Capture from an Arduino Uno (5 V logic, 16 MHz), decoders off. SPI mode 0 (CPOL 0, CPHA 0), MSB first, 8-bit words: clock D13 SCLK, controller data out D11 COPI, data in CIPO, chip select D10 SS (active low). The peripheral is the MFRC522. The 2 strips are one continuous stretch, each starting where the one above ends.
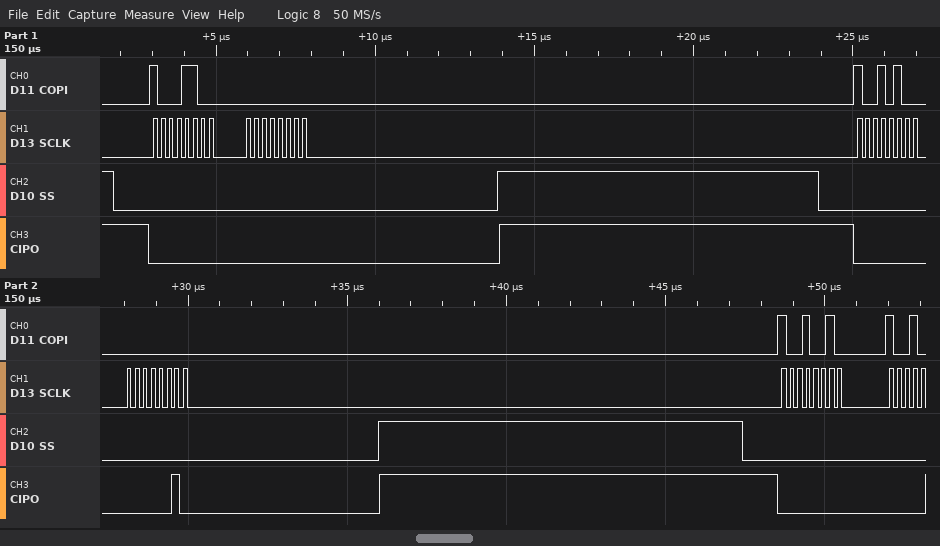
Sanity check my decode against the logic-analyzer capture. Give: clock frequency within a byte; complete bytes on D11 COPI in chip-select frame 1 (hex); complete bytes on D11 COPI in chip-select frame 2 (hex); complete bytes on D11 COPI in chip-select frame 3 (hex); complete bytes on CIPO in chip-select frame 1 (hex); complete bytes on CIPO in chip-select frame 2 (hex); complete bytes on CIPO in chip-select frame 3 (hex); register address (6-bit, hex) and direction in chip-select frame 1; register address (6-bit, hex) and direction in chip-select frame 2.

4 MHz
0x8C 0x00
0x94 0x00
0x92
0x00 0x00
0x00 0x02
0x00
0x06 read
0x0A read
